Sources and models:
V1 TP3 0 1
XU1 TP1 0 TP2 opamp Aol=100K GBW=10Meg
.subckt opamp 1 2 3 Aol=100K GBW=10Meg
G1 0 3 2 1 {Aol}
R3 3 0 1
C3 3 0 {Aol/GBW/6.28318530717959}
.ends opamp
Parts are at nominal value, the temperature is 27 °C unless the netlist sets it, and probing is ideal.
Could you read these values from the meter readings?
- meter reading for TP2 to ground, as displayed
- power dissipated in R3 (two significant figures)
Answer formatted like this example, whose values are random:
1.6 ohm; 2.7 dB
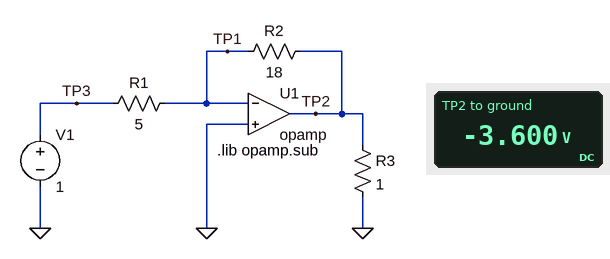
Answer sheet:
-3.600 V; 13 W
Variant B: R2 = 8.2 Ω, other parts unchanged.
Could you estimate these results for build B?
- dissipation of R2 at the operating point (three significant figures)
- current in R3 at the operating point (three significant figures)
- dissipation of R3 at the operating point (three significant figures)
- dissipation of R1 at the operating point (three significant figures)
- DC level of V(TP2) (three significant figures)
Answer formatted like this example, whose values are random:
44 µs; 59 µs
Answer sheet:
328 mW; 1.64 A; 2.69 W; 200 mW; -1.64 V
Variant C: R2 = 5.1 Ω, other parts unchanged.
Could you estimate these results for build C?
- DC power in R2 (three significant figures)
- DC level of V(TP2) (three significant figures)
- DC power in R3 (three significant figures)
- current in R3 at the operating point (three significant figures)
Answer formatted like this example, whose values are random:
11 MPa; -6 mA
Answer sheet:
204 mW; -1.02 V; 1.04 W; 1.02 A
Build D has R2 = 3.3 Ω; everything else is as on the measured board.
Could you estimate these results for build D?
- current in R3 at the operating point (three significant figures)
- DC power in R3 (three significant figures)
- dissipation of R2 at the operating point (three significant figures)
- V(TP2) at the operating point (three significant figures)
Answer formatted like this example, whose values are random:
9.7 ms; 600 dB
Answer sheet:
660 mA; 436 mW; 132 mW; -660 mV
